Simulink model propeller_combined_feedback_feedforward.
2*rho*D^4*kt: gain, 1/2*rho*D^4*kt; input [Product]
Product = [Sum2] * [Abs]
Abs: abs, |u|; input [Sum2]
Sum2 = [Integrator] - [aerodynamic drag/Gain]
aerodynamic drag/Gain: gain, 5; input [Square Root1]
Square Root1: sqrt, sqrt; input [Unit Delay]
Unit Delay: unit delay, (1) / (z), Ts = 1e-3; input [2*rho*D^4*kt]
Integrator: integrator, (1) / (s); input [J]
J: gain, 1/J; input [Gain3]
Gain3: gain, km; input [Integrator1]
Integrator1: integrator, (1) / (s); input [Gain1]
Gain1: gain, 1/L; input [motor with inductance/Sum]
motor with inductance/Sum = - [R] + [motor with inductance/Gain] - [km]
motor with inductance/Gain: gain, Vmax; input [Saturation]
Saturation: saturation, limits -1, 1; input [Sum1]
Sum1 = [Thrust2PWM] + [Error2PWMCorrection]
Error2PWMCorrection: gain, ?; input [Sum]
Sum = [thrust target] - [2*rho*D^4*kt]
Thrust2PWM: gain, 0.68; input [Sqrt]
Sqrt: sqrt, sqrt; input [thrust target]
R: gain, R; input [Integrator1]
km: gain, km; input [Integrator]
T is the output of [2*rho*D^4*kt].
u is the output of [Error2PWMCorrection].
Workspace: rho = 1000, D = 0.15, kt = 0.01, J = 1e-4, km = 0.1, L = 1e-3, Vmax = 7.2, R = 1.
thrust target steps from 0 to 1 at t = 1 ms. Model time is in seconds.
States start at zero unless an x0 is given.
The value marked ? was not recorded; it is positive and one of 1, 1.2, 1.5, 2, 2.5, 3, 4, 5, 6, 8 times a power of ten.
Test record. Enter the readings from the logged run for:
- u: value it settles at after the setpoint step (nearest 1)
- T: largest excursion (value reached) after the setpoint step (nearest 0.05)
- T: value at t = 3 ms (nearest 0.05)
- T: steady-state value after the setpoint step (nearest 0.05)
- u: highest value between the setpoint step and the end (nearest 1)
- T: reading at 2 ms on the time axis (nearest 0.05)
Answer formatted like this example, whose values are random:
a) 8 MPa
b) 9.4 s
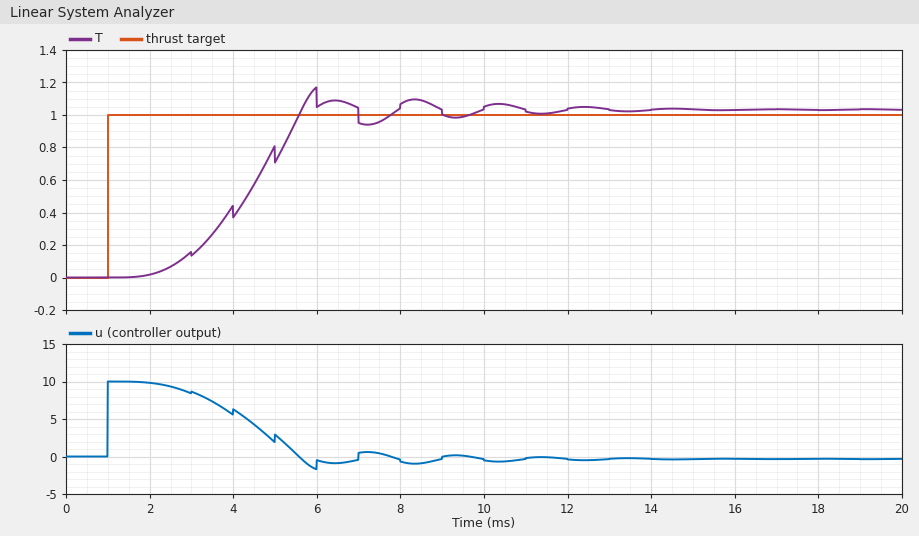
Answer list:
a) 0
b) 1.15
c) 0.15
d) 1.05
e) 10
f) 0.00
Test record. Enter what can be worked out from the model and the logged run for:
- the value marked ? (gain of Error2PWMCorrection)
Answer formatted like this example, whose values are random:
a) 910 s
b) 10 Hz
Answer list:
a) 10
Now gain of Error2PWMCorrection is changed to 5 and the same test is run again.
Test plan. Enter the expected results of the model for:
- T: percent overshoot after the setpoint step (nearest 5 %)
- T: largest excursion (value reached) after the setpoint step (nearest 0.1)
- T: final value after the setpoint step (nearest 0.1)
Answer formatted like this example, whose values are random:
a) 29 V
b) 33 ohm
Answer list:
a) 10 %
b) 1.2
c) 1.1
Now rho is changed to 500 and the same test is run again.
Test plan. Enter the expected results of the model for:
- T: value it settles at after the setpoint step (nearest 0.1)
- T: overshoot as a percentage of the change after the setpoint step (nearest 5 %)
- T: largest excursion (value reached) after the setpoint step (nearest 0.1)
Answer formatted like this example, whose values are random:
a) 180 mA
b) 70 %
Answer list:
a) 1.0
b) 10 %
c) 1.1
